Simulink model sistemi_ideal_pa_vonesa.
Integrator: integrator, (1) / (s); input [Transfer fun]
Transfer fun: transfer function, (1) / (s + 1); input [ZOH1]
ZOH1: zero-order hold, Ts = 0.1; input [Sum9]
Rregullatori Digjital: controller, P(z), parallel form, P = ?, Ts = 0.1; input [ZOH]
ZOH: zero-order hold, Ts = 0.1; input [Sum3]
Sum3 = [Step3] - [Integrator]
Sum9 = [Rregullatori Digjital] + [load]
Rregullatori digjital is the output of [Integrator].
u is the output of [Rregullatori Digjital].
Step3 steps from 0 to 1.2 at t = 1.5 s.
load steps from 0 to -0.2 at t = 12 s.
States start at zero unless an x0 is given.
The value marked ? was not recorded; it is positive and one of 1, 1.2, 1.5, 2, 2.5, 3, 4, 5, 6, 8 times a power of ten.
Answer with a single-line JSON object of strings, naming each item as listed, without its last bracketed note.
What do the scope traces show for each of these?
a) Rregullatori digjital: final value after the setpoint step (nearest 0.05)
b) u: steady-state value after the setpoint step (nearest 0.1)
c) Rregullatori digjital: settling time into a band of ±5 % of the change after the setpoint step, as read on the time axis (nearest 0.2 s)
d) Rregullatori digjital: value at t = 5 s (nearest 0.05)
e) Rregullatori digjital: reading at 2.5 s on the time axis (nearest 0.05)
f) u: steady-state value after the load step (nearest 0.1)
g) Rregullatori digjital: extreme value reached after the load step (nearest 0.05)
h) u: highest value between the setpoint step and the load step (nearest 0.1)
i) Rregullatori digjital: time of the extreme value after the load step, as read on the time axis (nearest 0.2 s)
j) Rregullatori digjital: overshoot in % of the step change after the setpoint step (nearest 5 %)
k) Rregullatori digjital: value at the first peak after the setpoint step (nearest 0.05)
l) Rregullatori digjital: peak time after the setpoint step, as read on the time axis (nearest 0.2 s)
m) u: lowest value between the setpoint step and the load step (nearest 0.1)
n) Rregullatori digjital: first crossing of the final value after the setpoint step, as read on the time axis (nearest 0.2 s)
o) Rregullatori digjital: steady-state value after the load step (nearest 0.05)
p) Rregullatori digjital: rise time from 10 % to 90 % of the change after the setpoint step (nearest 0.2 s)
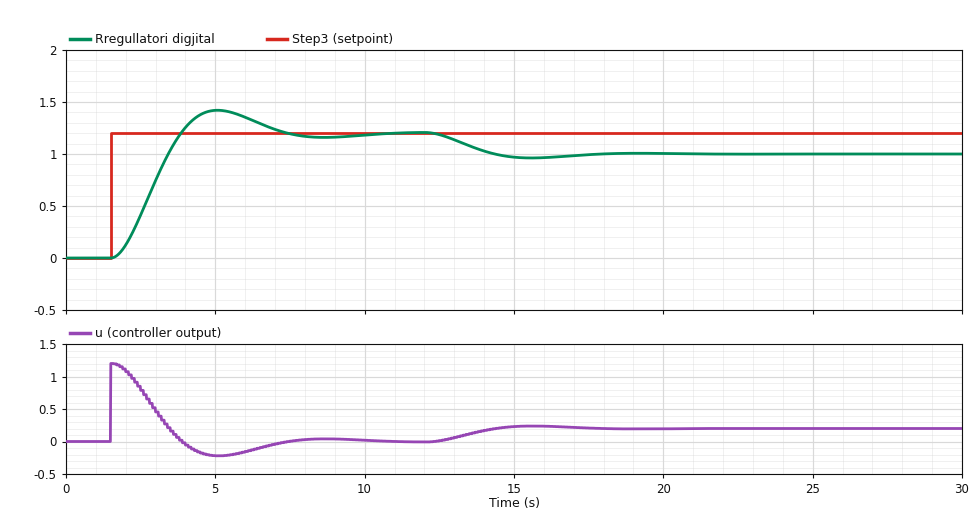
{"Rregullatori digjital: final value after the setpoint step": "1.20", "u: steady-state value after the setpoint step": "0.0", "Rregullatori digjital: settling time into a band of ±5 % of the change after the setpoint step, as read on the time axis": "6.8 s", "Rregullatori digjital: value at t = 5 s": "1.40", "Rregullatori digjital: reading at 2.5 s on the time axis": "0.40", "u: steady-state value after the load step": "0.2", "Rregullatori digjital: extreme value reached after the load step": "0.95", "u: highest value between the setpoint step and the load step": "1.2", "Rregullatori digjital: time of the extreme value after the load step, as read on the time axis": "15.6 s", "Rregullatori digjital: overshoot in % of the step change after the setpoint step": "20 %", "Rregullatori digjital: value at the first peak after the setpoint step": "1.40", "Rregullatori digjital: peak time after the setpoint step, as read on the time axis": "5.0 s", "u: lowest value between the setpoint step and the load step": "-0.2", "Rregullatori digjital: first crossing of the final value after the setpoint step, as read on the time axis": "3.8 s", "Rregullatori digjital: steady-state value after the load step": "1.00", "Rregullatori digjital: rise time from 10 % to 90 % of the change after the setpoint step": "1.6 s"}
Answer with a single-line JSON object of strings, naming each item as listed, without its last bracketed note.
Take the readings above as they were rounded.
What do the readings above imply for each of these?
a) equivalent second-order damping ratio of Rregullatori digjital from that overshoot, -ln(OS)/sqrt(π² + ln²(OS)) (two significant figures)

{"equivalent second-order damping ratio of Rregullatori digjital from that overshoot, -ln(OS)/sqrt(π² + ln²(OS))": "0.46"}
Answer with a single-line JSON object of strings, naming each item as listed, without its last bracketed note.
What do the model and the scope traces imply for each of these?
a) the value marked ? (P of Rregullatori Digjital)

{"the value marked ?": "1"}
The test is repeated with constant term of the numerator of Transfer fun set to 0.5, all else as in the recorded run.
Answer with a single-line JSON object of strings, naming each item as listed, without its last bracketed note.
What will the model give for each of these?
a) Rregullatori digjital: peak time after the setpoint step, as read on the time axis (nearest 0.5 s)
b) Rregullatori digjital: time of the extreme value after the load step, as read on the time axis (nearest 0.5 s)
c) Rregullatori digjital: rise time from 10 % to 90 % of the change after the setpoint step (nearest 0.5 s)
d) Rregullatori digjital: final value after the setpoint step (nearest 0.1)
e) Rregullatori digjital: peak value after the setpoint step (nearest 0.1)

{"Rregullatori digjital: peak time after the setpoint step, as read on the time axis": "7.5 s", "Rregullatori digjital: time of the extreme value after the load step, as read on the time axis": "18.0 s", "Rregullatori digjital: rise time from 10 % to 90 % of the change after the setpoint step": "3.0 s", "Rregullatori digjital: final value after the setpoint step": "1.2", "Rregullatori digjital: peak value after the setpoint step": "1.3"}
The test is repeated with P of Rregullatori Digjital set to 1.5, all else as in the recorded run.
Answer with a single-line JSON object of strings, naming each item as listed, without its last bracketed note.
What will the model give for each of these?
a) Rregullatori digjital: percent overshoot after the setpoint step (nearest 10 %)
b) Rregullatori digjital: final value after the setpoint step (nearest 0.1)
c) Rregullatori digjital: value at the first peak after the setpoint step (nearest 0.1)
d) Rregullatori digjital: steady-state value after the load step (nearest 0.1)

{"Rregullatori digjital: percent overshoot after the setpoint step": "30 %", "Rregullatori digjital: final value after the setpoint step": "1.2", "Rregullatori digjital: value at the first peak after the setpoint step": "1.5", "Rregullatori digjital: steady-state value after the load step": "1.1"}
